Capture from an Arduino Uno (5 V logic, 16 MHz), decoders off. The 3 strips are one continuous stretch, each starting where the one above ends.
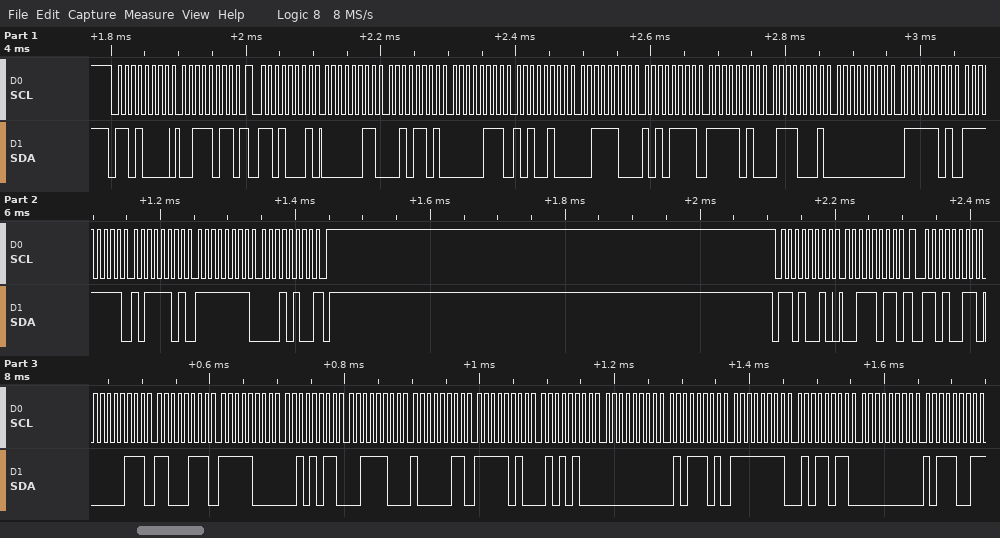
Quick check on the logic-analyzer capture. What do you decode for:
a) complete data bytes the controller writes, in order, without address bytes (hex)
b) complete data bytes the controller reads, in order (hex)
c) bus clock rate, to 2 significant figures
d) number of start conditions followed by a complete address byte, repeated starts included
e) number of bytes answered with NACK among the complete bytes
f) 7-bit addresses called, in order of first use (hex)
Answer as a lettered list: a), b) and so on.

a) 3B 3B
b) 03 2D 07 A4 3C AF FA 71 00 7D FF BD FF 14 07 C7 F8 2B 3C 83 FA 54 00 5D FF 5B 00 B9
c) 100 kHz
d) 4
e) 2
f) 0x68 0x69
